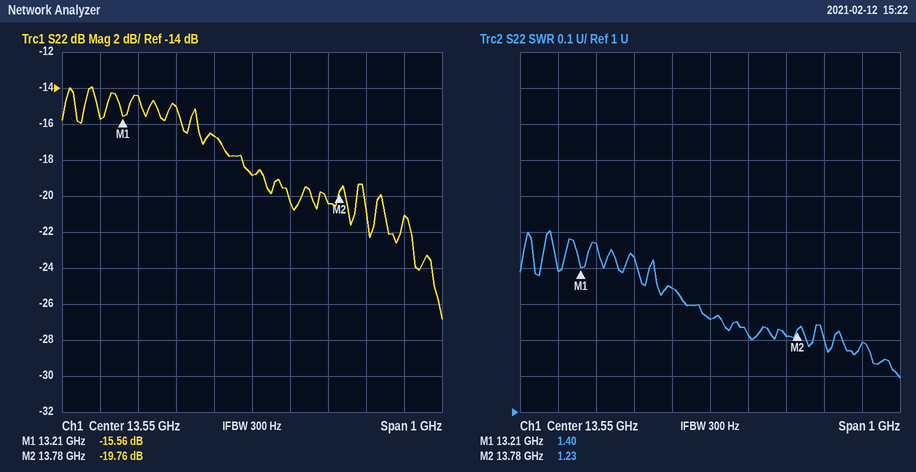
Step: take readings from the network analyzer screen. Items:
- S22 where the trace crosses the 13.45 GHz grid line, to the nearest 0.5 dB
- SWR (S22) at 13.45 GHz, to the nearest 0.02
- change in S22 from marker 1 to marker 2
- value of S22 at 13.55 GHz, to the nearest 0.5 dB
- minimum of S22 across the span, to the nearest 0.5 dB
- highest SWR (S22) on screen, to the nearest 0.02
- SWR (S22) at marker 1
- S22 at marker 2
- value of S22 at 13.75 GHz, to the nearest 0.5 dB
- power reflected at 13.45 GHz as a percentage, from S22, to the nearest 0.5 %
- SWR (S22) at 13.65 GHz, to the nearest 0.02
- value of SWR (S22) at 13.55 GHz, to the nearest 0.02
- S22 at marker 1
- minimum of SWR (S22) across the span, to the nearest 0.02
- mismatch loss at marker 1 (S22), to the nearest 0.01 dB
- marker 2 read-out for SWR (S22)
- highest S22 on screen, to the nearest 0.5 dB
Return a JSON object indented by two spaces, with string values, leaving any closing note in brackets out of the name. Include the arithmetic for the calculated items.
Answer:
{
  "S22 where the trace crosses the 13.45 GHz grid line, to the nearest 0.5 dB": "-16.5 dB",
  "SWR (S22) at 13.45 GHz, to the nearest 0.02": "1.34",
  "change in S22 from marker 1 to marker 2": "-19.76 − (-15.56) = -4.20 dB",
  "value of S22 at 13.55 GHz, to the nearest 0.5 dB": "-19.0 dB",
  "minimum of S22 across the span, to the nearest 0.5 dB": "-27.0 dB",
  "highest SWR (S22) on screen, to the nearest 0.02": "1.50",
  "SWR (S22) at marker 1": "1.40",
  "S22 at marker 2": "-19.76 dB",
  "value of S22 at 13.75 GHz, to the nearest 0.5 dB": "-20.5 dB",
  "power reflected at 13.45 GHz as a percentage, from S22, to the nearest 0.5 %": "10^(-16.5/10) ≈ 2.24 %, so 2.0 % to the nearest 0.5 %",
  "SWR (S22) at 13.65 GHz, to the nearest 0.02": "1.22",
  "value of SWR (S22) at 13.55 GHz, to the nearest 0.02": "1.26",
  "S22 at marker 1": "-15.56 dB",
  "minimum of SWR (S22) across the span, to the nearest 0.02": "1.10",
  "mismatch loss at marker 1 (S22), to the nearest 0.01 dB": "−10 log10(1 − 10^(-15.56/10)) ≈ 0.12 dB",
  "marker 2 read-out for SWR": "1.23",
  "highest S22 on screen, to the nearest 0.5 dB": "-14.0 dB"
}
